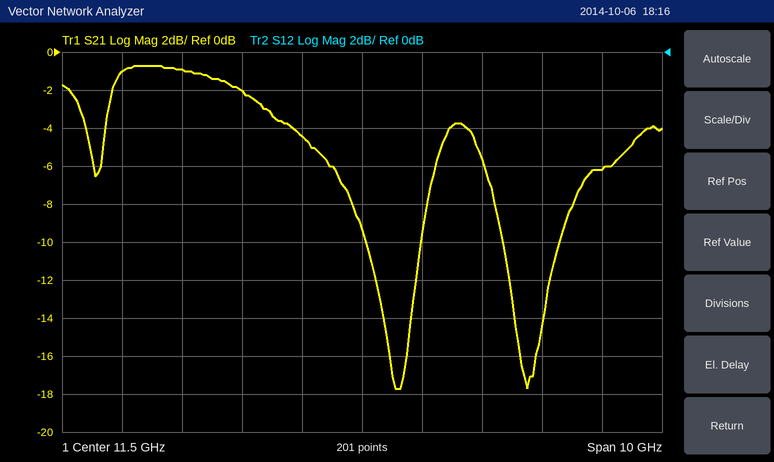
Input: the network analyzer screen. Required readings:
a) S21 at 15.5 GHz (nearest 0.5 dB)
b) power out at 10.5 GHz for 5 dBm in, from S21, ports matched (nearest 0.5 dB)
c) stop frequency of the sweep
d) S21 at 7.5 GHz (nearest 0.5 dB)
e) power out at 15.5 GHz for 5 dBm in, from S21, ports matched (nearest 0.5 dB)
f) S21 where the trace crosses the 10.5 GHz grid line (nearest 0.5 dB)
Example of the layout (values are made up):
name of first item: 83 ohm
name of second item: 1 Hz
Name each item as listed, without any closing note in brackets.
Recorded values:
S21 at 15.5 GHz: -6.0 dB
power out at 10.5 GHz for 5 dBm in, from S21, ports matched: 0.5 dBm
stop frequency of the sweep: 16.5 GHz
S21 at 7.5 GHz: -1.0 dB
power out at 15.5 GHz for 5 dBm in, from S21, ports matched: -1.0 dBm
S21 where the trace crosses the 10.5 GHz grid line: -4.5 dB
